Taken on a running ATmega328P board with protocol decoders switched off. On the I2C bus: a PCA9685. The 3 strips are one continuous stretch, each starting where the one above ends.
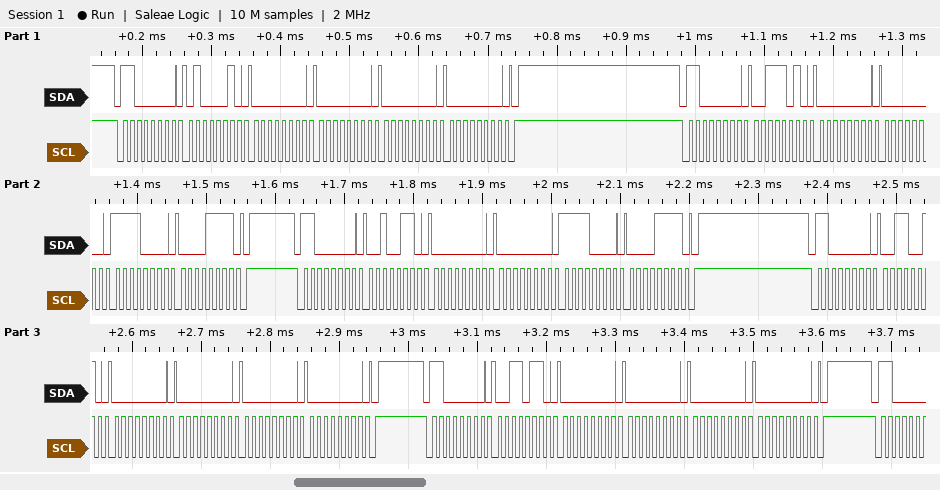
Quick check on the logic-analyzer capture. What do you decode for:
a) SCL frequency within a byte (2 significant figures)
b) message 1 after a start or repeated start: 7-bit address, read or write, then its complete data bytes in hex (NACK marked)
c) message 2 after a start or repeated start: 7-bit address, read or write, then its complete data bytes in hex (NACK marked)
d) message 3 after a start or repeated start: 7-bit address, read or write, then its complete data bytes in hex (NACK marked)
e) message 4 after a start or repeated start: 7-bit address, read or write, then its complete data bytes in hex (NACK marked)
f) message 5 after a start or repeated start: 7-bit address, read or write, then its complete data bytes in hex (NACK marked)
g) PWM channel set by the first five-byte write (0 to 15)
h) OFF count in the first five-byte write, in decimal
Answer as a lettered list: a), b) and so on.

a) 100 kHz
b) 0x60 write: 42 00 00 00 00
c) 0x60 write: 3A 00 00 F0 0F
d) 0x60 write: 26 00 00 F0 0F
e) 0x60 write: 32 00 00 00 00
f) 0x60 write: 36 00 00 00 00
g) 15
h) 0
